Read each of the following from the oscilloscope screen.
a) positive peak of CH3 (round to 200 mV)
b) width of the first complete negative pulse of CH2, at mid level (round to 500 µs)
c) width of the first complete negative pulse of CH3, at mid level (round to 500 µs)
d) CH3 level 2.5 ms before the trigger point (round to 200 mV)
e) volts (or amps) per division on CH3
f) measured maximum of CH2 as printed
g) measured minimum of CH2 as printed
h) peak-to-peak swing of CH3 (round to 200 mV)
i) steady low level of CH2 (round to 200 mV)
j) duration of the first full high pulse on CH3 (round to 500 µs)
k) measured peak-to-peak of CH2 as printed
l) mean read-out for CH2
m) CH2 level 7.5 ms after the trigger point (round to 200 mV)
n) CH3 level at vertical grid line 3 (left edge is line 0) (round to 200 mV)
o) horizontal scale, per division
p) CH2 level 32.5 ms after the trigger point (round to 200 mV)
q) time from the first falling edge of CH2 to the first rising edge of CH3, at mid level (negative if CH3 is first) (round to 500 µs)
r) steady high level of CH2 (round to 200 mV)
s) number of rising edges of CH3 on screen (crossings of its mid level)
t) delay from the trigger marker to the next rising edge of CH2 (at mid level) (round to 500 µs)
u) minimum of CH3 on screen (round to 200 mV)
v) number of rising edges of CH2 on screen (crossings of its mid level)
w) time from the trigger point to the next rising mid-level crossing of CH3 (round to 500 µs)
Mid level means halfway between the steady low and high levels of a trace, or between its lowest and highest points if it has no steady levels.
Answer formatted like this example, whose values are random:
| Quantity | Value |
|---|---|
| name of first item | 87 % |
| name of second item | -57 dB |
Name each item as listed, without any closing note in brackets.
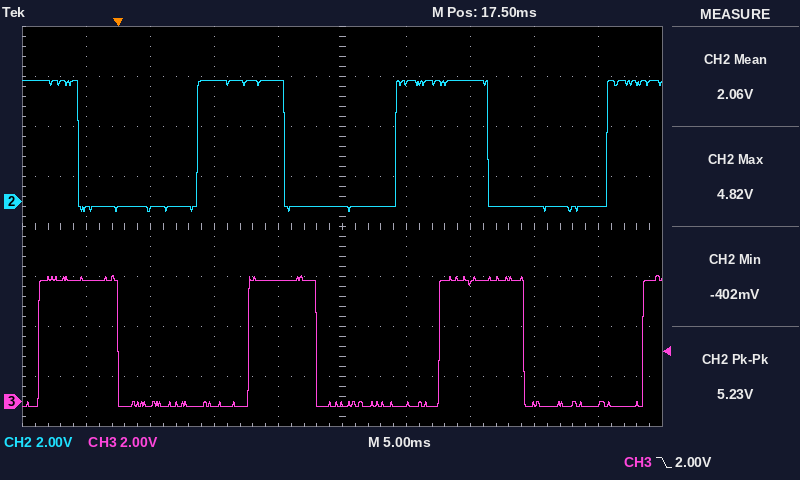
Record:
| Quantity | Value |
|---|---|
| positive peak of CH3 | 5.0 V |
| width of the first complete negative pulse of CH2, at mid level | 9.5 ms |
| width of the first complete negative pulse of CH3, at mid level | 10.0 ms |
| CH3 level 2.5 ms before the trigger point | 4.8 V |
| volts (or amps) per division on CH3 | 2 V |
| measured maximum of CH2 as printed | 4.82 V |
| measured minimum of CH2 as printed | -402 mV |
| peak-to-peak swing of CH3 | 5.2 V |
| steady low level of CH2 | -200 mV |
| duration of the first full high pulse on CH3 | 6.0 ms |
| measured peak-to-peak of CH2 as printed | 5.23 V |
| mean read-out for CH2 | 2.06 V |
| CH2 level 7.5 ms after the trigger point | 4.8 V |
| CH3 level at vertical grid line 3 (left edge is line 0) | -200 mV |
| horizontal scale, per division | 5 ms |
| CH2 level 32.5 ms after the trigger point | -200 mV |
| time from the first falling edge of CH2 to the first rising edge of CH3, at mid level (negative if CH3 is first) | -3.0 ms |
| steady high level of CH2 | 4.8 V |
| number of rising edges of CH3 on screen | 4 |
| delay from the trigger marker to the next rising edge of CH2 (at mid level) | 6.0 ms |
| minimum of CH3 on screen | -200 mV |
| number of rising edges of CH2 on screen | 3 |
| time from the trigger point to the next rising mid-level crossing of CH3 | 10.0 ms |
